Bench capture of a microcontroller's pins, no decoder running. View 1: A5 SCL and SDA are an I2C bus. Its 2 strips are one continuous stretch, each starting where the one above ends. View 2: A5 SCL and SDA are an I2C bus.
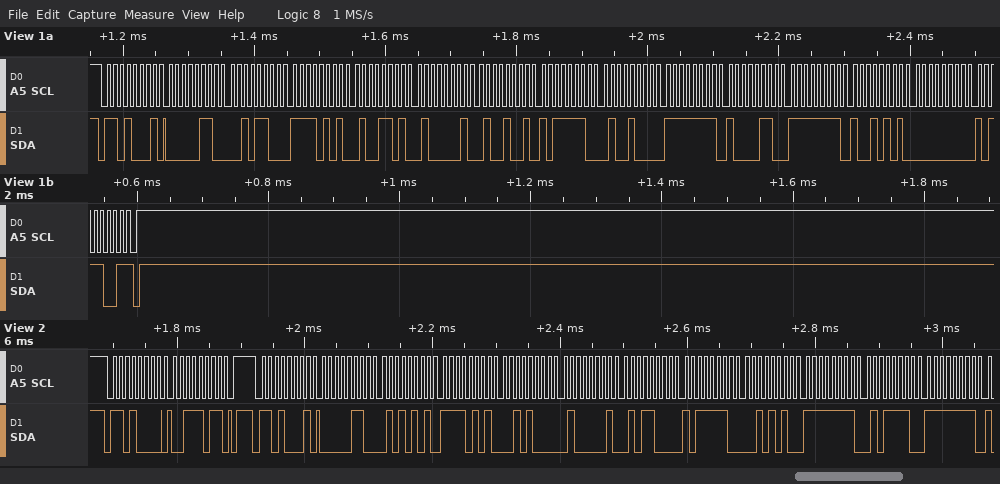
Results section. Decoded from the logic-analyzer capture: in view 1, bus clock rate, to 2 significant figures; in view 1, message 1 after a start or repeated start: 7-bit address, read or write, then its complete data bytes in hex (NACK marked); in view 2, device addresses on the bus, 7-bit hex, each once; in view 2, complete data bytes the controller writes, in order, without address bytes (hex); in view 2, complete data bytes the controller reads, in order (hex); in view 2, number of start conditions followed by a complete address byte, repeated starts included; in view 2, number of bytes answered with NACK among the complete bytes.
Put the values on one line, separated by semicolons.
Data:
100 kHz; 0x68 read: 06 2C F5 4D 41 49 BE 48 FF 86 FF 95 00 B9 NACK; 0x68; 3B; 06 55 F5 28 41 58 BE 2A FF 5E FF; 2; 0
